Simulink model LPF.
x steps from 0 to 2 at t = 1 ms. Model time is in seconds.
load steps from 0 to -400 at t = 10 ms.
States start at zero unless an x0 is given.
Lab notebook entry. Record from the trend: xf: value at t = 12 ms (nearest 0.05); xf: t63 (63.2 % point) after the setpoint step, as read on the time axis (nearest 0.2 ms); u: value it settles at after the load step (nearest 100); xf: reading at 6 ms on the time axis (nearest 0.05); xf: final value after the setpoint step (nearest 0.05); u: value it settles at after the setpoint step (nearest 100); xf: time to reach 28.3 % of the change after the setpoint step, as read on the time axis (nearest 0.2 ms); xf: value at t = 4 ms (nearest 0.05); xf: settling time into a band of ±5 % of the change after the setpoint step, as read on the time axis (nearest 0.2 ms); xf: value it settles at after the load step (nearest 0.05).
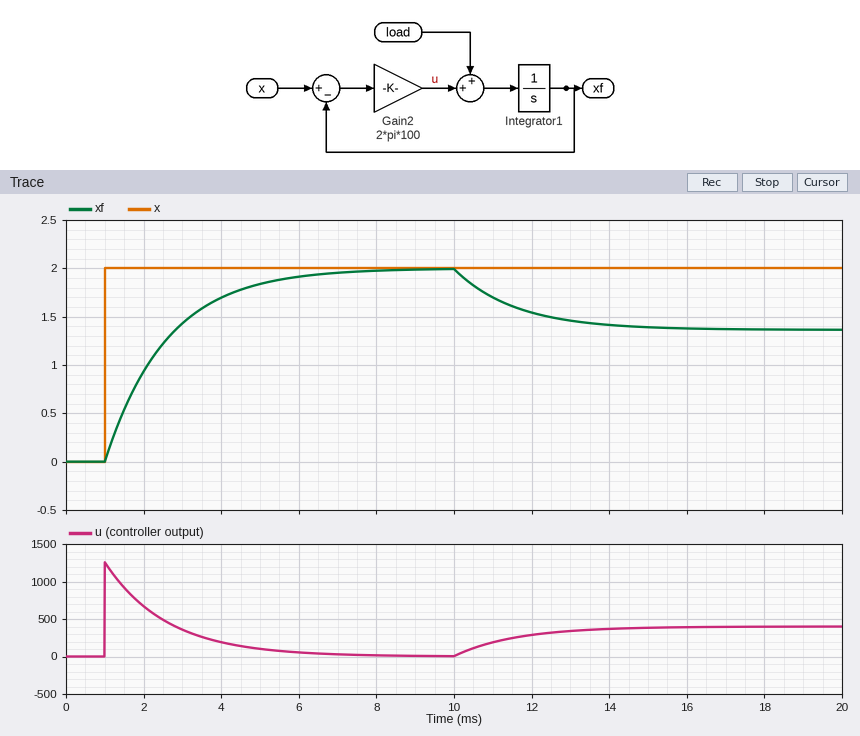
1.55
2.6 ms
400
1.90
2.00
0
1.6 ms
1.70
5.8 ms
1.35
